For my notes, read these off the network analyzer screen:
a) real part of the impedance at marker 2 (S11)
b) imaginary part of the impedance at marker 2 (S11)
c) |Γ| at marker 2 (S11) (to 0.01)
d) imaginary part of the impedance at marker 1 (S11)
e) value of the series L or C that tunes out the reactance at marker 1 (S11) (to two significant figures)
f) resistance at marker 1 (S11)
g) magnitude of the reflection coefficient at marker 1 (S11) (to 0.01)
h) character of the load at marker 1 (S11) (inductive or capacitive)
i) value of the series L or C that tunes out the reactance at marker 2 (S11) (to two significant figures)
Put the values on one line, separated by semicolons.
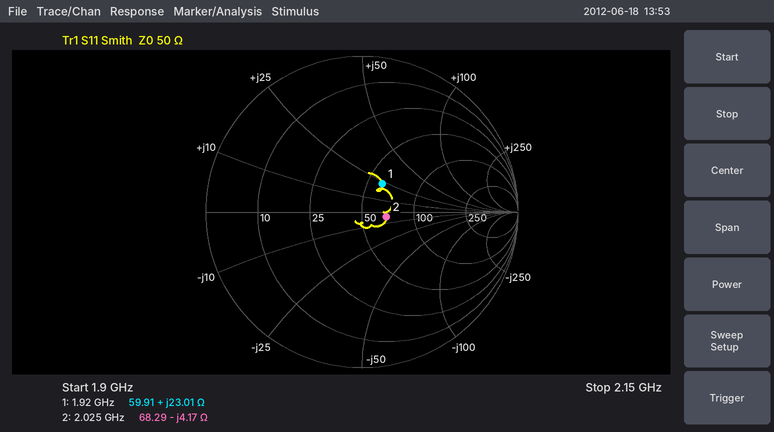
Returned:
68.29 Ω; -4.17 Ω; 0.16; +23.01 Ω; 3.6 pF; 59.91 Ω; 0.22; inductive; 330 pH
